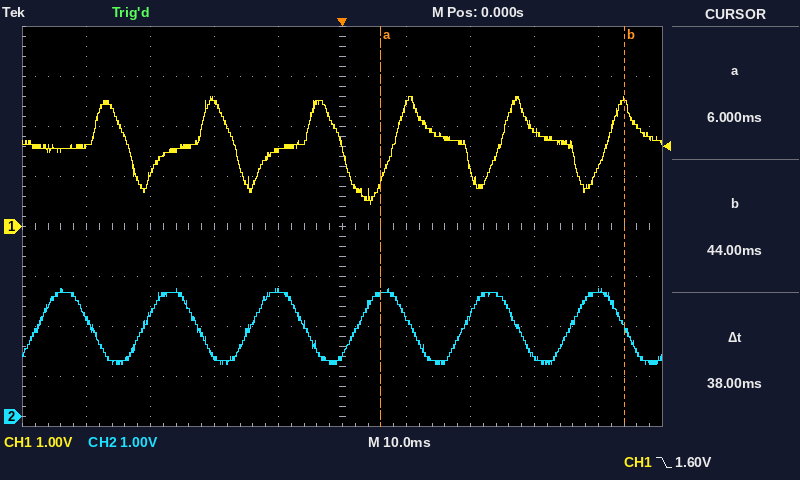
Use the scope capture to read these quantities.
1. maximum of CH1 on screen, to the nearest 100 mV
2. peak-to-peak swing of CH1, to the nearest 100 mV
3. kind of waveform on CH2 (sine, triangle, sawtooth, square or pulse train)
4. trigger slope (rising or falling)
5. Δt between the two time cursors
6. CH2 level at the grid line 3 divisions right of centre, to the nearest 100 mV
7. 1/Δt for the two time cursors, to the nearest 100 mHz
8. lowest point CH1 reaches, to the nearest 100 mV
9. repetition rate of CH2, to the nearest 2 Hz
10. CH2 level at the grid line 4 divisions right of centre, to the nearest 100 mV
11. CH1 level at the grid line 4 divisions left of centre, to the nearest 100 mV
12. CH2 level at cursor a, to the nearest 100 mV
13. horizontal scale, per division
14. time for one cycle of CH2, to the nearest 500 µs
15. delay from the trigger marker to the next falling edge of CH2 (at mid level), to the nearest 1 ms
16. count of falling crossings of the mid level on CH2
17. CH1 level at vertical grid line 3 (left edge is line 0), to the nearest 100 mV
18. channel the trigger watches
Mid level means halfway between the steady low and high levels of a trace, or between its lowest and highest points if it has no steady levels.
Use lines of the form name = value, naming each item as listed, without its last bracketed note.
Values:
maximum of CH1 on screen, to the nearest 100 mV = 2.6 V
peak-to-peak swing of CH1, to the nearest 100 mV = 2.2 V
kind of waveform on CH2 = sine
trigger slope = falling
Δt between the two time cursors = 38 ms
CH2 level at the grid line 3 divisions right of centre, to the nearest 100 mV = 1.2 V
1/Δt for the two time cursors, to the nearest 100 mHz = 26.3 Hz
lowest point CH1 reaches, to the nearest 100 mV = 400 mV
repetition rate of CH2, to the nearest 2 Hz = 60 Hz
CH2 level at the grid line 4 divisions right of centre, to the nearest 100 mV = 2.5 V
CH1 level at the grid line 4 divisions left of centre, to the nearest 100 mV = 1.6 V
CH2 level at cursor a, to the nearest 100 mV = 2.4 V
horizontal scale, per division = 10 ms
time for one cycle of CH2, to the nearest 500 µs = 16.5 ms
delay from the trigger marker to the next falling edge of CH2 (at mid level), to the nearest 1 ms = 11 ms
count of falling crossings of the mid level on CH2 = 6
CH1 level at vertical grid line 3 (left edge is line 0), to the nearest 100 mV = 2.5 V
channel the trigger watches = CH1
